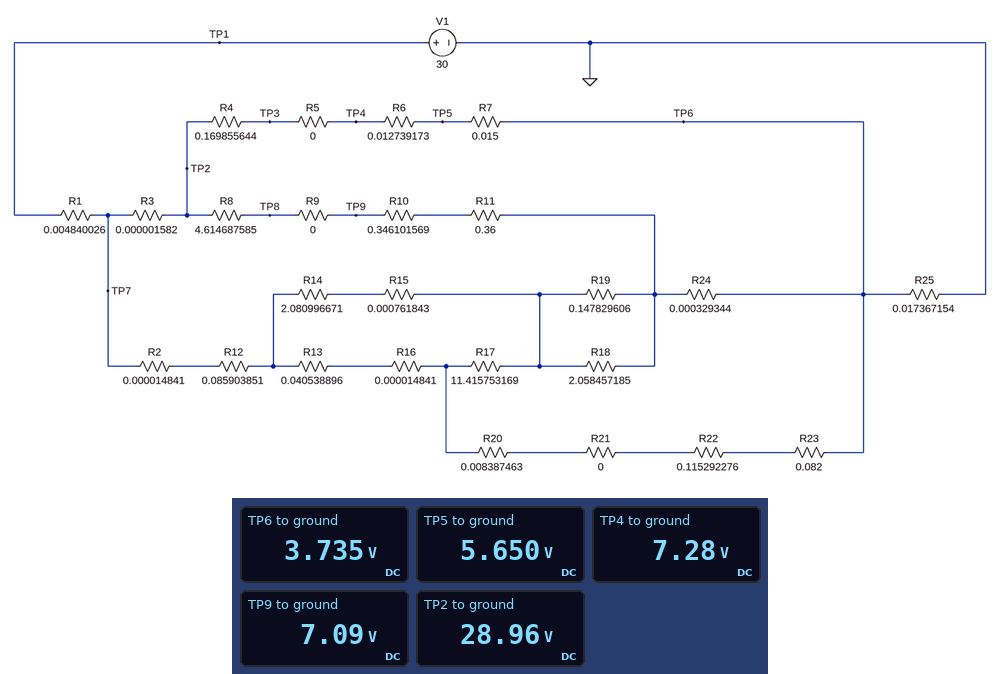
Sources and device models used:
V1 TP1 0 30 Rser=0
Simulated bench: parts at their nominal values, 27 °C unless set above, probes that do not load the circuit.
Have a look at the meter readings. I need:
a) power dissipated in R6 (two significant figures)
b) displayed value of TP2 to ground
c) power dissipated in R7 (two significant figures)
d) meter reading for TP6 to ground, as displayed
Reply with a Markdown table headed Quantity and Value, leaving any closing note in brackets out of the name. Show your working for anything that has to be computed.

| Quantity | Value |
|---|---|
| power dissipated in R6 | (7.28 V - 5.65 V)^2 / 12.74 mΩ = 210 W |
| displayed value of TP2 to ground | 28.96 V |
| power dissipated in R7 | (5.65 V - 3.735 V)^2 / 15 mΩ = 240 W |
| meter reading for TP6 to ground, as displayed | 3.735 V |
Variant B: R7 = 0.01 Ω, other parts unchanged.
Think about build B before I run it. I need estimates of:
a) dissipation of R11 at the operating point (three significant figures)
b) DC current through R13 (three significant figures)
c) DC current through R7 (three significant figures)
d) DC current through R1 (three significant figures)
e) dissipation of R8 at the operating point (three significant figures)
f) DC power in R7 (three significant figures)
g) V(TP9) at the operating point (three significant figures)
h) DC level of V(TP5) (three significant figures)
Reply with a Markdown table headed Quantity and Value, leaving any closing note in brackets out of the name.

| Quantity | Value |
|---|---|
| dissipation of R11 at the operating point | 8.05 W |
| DC current through R13 | 74.4 A |
| DC current through R7 | 131 A |
| DC current through R1 | 218 A |
| dissipation of R8 at the operating point | 103 W |
| DC power in R7 | 171 W |
| V(TP9) at the operating point | 7.13 V |
| DC level of V(TP5) | 5.09 V |
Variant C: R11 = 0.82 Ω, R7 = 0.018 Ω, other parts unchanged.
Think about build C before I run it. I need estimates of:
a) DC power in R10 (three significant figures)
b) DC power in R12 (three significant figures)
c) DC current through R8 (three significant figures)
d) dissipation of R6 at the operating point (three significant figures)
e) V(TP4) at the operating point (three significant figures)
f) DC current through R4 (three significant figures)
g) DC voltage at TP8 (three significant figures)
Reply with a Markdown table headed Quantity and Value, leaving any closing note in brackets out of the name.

| Quantity | Value |
|---|---|
| DC power in R10 | 6.61 W |
| DC power in R12 | 589 W |
| DC current through R8 | 4.37 A |
| dissipation of R6 at the operating point | 202 W |
| V(TP4) at the operating point | 7.57 V |
| DC current through R4 | 126 A |
| DC voltage at TP8 | 8.80 V |
